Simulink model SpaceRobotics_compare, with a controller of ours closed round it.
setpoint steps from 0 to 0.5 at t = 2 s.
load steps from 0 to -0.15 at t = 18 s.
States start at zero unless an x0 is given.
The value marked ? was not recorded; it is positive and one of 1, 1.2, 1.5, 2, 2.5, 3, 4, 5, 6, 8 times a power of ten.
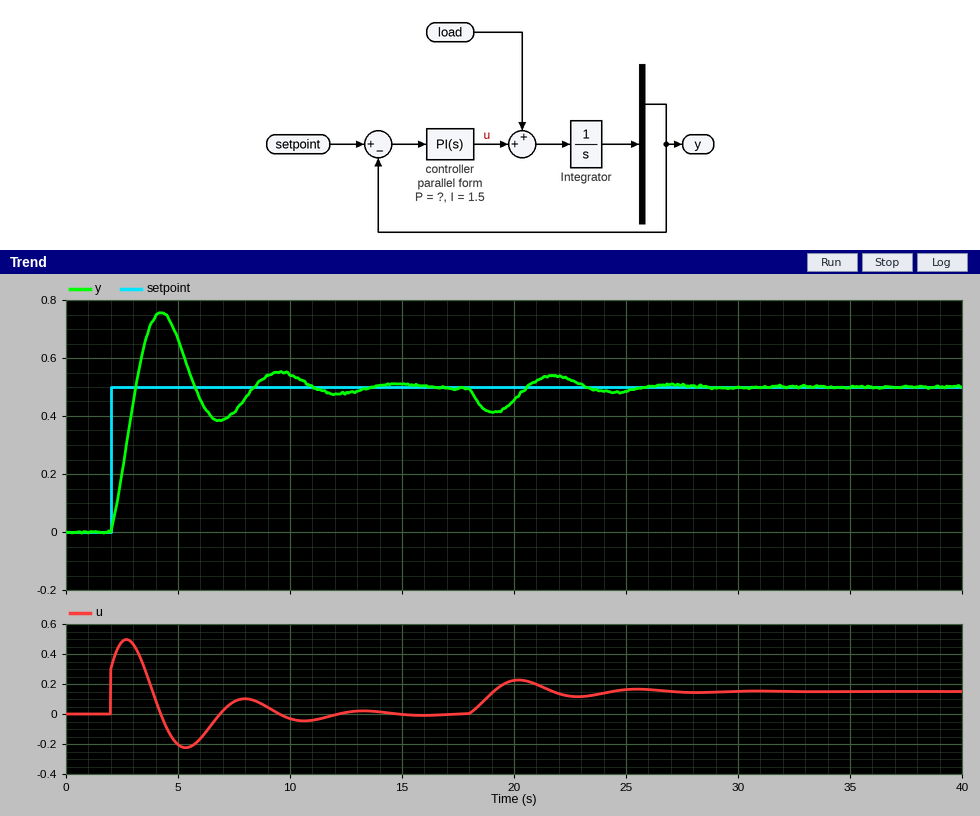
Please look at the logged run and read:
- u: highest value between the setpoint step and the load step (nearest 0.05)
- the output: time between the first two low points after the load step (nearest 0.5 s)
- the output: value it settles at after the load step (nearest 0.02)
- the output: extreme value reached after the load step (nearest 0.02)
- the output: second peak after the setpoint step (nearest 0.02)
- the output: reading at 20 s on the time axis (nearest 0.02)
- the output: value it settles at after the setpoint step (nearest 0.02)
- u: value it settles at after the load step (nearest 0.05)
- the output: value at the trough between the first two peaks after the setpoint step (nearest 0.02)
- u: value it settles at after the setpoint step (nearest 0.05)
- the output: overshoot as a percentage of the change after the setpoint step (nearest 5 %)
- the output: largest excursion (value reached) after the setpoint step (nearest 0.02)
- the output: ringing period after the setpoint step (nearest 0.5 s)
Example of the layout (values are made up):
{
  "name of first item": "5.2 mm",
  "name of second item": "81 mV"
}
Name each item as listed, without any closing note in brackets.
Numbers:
{
  "u: highest value between the setpoint step and the load step": "0.50",
  "the output: time between the first two low points after the load step": "5.5 s",
  "the output: value it settles at after the load step": "0.50",
  "the output: extreme value reached after the load step": "0.42",
  "the output: second peak after the setpoint step": "0.56",
  "the output: reading at 20 s on the time axis": "0.46",
  "the output: value it settles at after the setpoint step": "0.50",
  "u: value it settles at after the load step": "0.15",
  "the output: value at the trough between the first two peaks after the setpoint step": "0.38",
  "u: value it settles at after the setpoint step": "0.00",
  "the output: overshoot as a percentage of the change after the setpoint step": "50 %",
  "the output: largest excursion (value reached) after the setpoint step": "0.76",
  "the output: ringing period after the setpoint step": "5.5 s"
}
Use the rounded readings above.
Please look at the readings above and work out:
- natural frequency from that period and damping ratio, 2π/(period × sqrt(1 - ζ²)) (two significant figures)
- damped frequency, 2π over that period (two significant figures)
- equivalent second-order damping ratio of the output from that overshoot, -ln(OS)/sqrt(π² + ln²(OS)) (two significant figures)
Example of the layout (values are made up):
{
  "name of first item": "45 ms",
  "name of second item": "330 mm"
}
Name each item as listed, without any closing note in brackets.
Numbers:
{
  "natural frequency from that period and damping ratio, 2π/(period × sqrt(1 - ζ²))": "1.2 rad/s",
  "damped frequency, 2π over that period": "1.1 rad/s",
  "equivalent second-order damping ratio of the output from that overshoot, -ln(OS)/sqrt(π² + ln²(OS))": "0.22"
}
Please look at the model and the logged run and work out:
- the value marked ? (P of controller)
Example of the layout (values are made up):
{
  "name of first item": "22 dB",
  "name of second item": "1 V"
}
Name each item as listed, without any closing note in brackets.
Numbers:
{
  "the value marked ?": "0.6"
}
